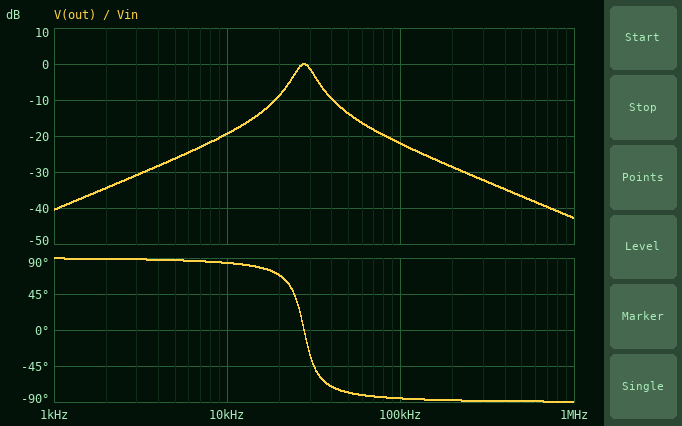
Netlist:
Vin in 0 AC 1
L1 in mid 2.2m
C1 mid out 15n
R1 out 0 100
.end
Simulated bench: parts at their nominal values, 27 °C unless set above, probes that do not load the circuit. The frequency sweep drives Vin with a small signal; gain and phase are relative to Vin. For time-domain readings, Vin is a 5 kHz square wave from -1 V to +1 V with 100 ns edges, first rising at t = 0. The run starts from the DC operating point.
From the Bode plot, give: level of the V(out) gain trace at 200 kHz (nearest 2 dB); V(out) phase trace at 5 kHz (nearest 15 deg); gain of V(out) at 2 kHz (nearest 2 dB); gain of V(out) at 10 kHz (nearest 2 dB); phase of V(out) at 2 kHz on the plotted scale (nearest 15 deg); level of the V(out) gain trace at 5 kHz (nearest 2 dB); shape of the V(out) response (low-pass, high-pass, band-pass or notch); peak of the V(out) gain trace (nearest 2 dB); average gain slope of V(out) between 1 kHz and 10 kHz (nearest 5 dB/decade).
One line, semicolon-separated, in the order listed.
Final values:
-28 dB; 90 deg; -34 dB; -20 dB; 90 deg; -26 dB; band-pass; 0 dB; 20 dB/decade
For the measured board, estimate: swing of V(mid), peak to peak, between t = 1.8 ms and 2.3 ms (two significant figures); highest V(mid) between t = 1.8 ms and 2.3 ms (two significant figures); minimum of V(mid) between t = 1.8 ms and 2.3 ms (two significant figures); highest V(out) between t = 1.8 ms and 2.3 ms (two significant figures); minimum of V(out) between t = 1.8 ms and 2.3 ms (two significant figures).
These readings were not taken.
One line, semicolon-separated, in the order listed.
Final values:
4.8 V; 2.4 V; -2.4 V; 440 mV; -440 mV
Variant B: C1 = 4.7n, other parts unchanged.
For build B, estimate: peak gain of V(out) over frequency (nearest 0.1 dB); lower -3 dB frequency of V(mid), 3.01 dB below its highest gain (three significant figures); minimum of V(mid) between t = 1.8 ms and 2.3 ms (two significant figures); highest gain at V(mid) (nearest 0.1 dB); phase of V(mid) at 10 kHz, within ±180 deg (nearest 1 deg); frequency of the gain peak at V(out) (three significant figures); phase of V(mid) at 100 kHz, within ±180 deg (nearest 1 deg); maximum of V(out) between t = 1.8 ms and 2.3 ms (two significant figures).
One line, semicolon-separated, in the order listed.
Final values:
0 dB; 45.5 kHz; -2.5 V; 16.8 dB; 0 deg; 49.5 kHz; -158 deg; 240 mV
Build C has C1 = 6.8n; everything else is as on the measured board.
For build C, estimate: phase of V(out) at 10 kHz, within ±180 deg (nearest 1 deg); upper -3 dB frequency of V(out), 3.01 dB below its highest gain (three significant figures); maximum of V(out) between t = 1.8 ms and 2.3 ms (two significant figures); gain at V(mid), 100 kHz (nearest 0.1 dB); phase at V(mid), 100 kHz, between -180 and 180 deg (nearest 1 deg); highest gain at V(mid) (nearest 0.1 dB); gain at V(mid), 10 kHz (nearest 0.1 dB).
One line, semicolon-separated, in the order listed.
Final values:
87 deg; 44.9 kHz; 280 mV; -13.1 dB; -152 deg; 15.3 dB; 0.5 dB
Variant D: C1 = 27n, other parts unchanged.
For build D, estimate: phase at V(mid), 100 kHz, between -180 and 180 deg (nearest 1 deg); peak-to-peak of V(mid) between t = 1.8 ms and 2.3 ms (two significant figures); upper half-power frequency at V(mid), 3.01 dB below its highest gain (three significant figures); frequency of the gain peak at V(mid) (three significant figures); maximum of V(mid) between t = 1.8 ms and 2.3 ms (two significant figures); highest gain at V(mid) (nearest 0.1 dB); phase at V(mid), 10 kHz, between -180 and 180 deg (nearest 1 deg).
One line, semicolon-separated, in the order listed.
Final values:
-116 deg; 4.2 V; 23.5 kHz; 20.1 kHz; 2.1 V; 9.7 dB; -3 deg
